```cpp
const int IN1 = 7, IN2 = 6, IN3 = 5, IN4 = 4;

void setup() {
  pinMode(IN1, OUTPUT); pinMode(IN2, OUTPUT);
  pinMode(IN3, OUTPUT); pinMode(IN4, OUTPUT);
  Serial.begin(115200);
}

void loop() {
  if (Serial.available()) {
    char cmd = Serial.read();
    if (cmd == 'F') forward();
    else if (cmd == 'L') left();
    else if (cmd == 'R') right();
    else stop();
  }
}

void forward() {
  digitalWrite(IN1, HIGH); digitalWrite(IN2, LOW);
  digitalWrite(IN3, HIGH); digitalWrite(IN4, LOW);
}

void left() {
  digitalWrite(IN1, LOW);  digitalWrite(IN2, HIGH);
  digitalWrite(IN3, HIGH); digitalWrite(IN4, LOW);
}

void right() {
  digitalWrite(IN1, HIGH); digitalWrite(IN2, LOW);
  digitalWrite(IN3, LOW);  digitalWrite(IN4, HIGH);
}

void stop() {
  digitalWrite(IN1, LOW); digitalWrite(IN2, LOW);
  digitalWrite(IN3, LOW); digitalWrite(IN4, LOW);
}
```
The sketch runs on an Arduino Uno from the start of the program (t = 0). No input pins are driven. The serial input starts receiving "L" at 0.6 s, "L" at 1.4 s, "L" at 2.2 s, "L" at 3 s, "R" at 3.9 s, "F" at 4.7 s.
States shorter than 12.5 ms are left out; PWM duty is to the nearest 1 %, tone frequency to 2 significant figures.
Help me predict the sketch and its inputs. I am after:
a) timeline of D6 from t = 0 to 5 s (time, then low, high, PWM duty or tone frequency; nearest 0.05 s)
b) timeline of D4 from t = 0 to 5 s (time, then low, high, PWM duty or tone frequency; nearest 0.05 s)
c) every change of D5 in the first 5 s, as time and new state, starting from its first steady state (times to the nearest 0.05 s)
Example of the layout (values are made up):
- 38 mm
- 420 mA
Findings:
- 0 s low; 0.6 s high; 3.9 s low
- 0 s low; 3.9 s high; 4.7 s low
- 0 s low; 0.6 s high; 3.9 s low; 4.7 s high
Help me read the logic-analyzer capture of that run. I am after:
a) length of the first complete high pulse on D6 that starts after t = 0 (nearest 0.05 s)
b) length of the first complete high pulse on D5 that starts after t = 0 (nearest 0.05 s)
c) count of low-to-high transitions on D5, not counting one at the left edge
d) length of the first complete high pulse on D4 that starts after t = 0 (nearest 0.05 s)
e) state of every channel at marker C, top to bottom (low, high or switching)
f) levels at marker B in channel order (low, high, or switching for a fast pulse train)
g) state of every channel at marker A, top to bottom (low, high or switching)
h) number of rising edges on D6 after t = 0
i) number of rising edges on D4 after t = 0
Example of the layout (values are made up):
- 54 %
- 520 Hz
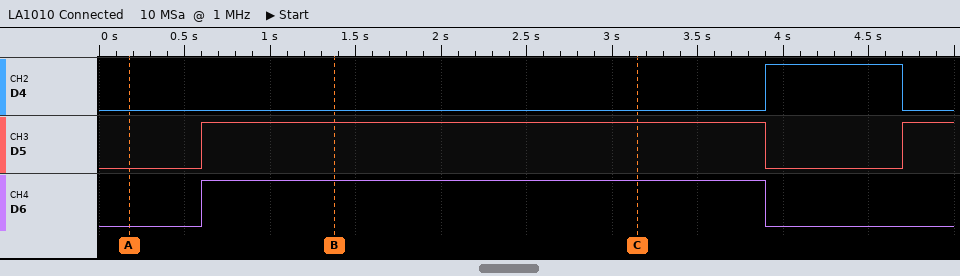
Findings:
- 3.30 s
- 3.30 s
- 2
- 0.80 s
- D4 low, D5 high, D6 high
- D4 low, D5 high, D6 high
- D4 low, D5 low, D6 low
- 1
- 1
